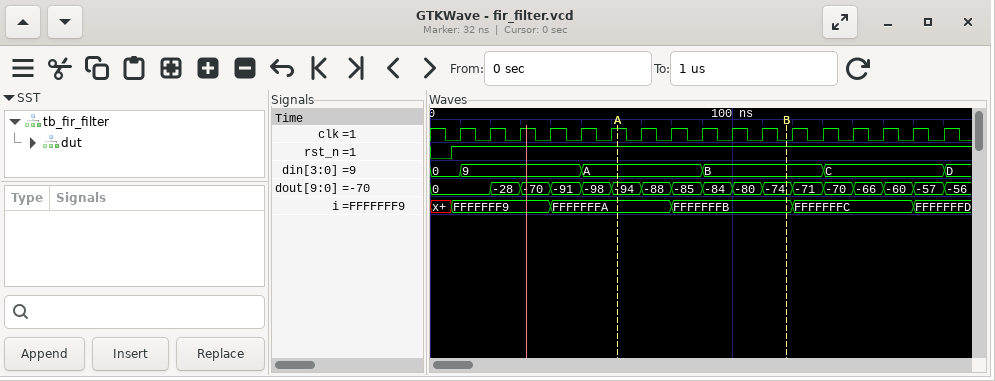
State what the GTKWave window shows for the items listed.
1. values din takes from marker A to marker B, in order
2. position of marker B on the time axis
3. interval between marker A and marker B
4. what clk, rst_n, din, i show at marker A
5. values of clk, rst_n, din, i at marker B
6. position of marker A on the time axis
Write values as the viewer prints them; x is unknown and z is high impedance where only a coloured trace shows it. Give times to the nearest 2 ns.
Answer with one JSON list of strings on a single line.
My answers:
["A, B", "118 ns", "56 ns", "clk=1, rst_n=1, din=A, i=FFFFFFFA", "clk=0, rst_n=1, din=B, i=FFFFFFFB", "62 ns"]
